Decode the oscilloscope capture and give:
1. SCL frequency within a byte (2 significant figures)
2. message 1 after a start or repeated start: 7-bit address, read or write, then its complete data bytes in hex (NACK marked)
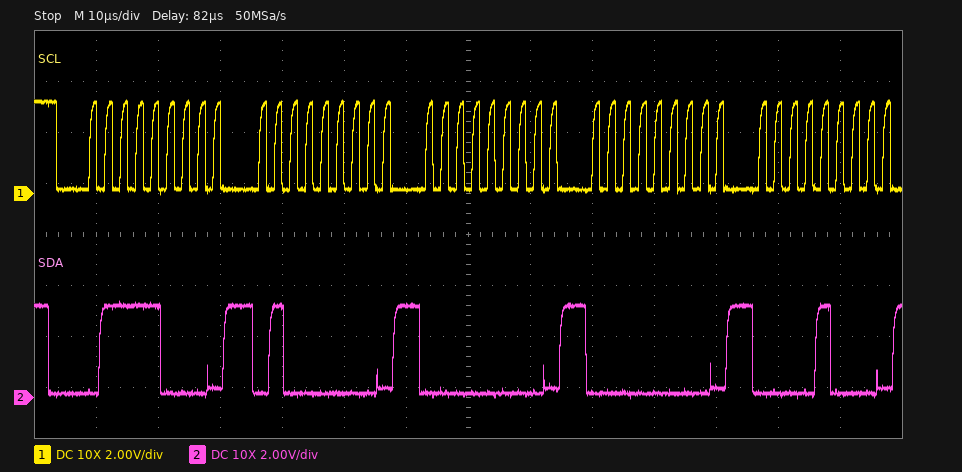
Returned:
400 kHz
0x3C write: 40 00 00 08
